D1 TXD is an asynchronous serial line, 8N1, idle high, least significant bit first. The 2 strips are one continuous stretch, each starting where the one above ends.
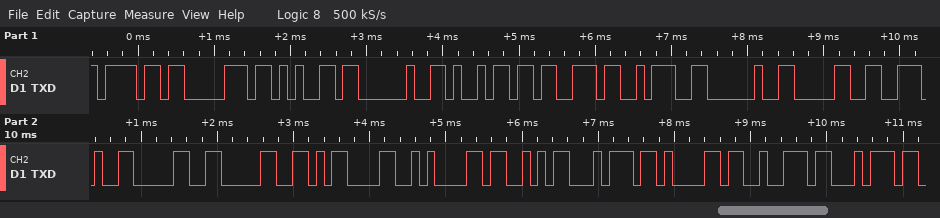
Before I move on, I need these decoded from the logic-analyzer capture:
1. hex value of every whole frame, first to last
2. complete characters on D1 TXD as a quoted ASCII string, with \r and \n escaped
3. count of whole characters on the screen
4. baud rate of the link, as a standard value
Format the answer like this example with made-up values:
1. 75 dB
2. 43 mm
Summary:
1. 6F 70 65 20 69 73 3A 20 30 2E 30 30 0D 0A 53 74 61 72 74
2. "ope is: 0.00\r\nStart"
3. 19
4. 9600 baud
